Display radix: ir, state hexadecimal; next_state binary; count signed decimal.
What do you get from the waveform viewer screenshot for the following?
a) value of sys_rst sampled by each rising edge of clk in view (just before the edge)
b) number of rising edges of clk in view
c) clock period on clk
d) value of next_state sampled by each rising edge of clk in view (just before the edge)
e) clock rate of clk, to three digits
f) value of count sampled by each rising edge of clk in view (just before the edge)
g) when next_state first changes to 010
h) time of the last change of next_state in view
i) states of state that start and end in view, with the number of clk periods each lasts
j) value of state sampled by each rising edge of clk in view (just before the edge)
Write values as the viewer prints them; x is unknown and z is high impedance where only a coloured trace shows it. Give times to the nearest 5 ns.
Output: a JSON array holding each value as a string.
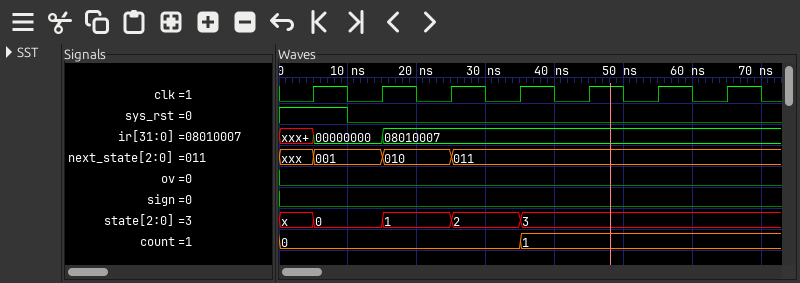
["1 0 0 0 0 0 0", "7", "10 ns", "xxx, 001, 010, 011, 011, 011, 011", "100 MHz", "0, 0, 0, 0, 1, 1, 1", "15 ns", "25 ns", "0: 1, 1: 1, 2: 1", "x, 0, 1, 2, 3, 3, 3"]
